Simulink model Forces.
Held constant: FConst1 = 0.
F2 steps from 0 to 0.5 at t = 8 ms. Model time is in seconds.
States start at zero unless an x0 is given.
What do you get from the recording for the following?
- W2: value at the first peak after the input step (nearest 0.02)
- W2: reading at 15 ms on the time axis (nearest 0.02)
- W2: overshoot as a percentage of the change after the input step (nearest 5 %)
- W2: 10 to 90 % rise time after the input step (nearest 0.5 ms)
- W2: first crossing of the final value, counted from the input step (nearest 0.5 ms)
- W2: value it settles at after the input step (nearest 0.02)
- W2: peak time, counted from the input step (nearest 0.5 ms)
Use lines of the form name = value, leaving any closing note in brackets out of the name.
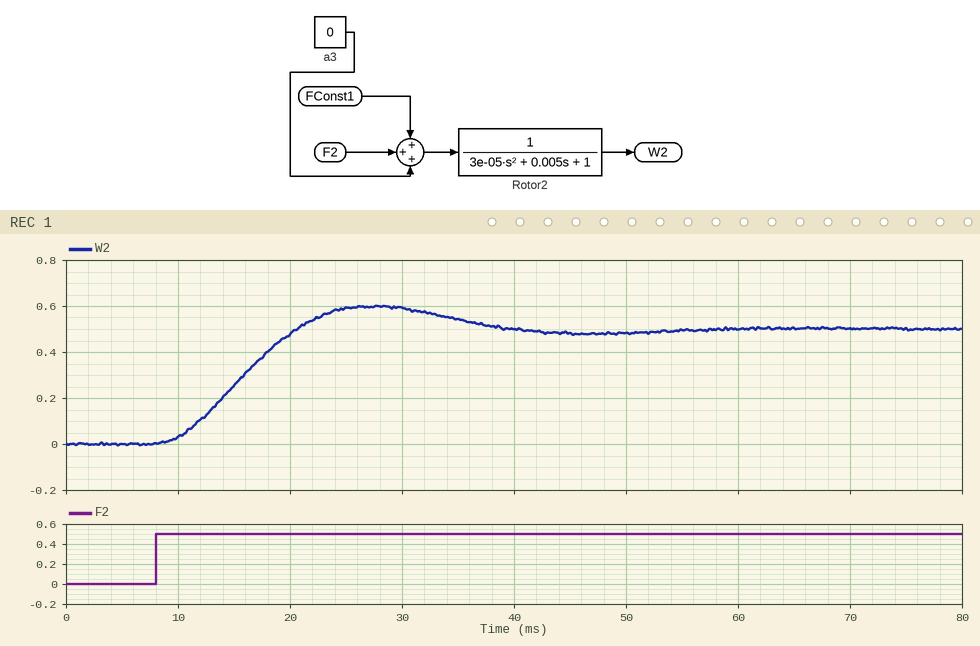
W2: value at the first peak after the input step = 0.60
W2: reading at 15 ms on the time axis = 0.26
W2: overshoot as a percentage of the change after the input step = 20 %
W2: 10 to 90 % rise time after the input step = 8.5 ms
W2: first crossing of the final value, counted from the input step = 12.5 ms
W2: value it settles at after the input step = 0.50
W2: peak time, counted from the input step = 19.5 ms
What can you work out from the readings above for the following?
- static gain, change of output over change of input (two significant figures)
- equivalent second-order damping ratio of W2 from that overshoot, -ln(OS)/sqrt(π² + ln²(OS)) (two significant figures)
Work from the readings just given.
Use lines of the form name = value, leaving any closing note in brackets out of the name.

static gain, change of output over change of input = 1.0
equivalent second-order damping ratio of W2 from that overshoot, -ln(OS)/sqrt(π² + ln²(OS)) = 0.46
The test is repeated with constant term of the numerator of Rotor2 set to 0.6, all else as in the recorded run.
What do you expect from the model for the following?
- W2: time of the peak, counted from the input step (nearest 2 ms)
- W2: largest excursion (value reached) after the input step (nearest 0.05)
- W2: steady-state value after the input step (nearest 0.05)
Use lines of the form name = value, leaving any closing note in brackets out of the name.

W2: time of the peak, counted from the input step = 20 ms
W2: largest excursion (value reached) after the input step = 0.35
W2: steady-state value after the input step = 0.30
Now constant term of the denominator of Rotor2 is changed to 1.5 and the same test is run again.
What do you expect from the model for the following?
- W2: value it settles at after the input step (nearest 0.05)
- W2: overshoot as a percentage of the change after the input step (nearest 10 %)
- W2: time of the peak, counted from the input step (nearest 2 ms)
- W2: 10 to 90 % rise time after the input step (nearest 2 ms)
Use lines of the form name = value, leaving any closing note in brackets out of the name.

W2: value it settles at after the input step = 0.35
W2: overshoot as a percentage of the change after the input step = 30 %
W2: time of the peak, counted from the input step = 16 ms
W2: 10 to 90 % rise time after the input step = 6 ms
